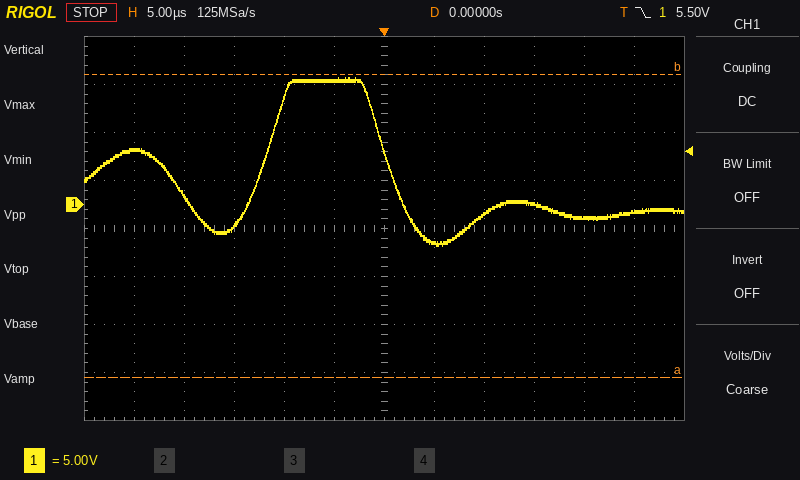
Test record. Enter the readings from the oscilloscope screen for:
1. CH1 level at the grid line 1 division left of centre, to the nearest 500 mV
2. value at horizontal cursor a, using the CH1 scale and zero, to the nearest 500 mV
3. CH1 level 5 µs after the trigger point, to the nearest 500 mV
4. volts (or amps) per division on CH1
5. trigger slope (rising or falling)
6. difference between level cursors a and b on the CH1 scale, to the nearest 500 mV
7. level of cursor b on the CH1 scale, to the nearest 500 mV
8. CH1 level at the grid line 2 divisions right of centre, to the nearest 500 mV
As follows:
13.0 V
-18.0 V
-4.0 V
5 V
falling
31.5 V
13.5 V
-1.0 V
